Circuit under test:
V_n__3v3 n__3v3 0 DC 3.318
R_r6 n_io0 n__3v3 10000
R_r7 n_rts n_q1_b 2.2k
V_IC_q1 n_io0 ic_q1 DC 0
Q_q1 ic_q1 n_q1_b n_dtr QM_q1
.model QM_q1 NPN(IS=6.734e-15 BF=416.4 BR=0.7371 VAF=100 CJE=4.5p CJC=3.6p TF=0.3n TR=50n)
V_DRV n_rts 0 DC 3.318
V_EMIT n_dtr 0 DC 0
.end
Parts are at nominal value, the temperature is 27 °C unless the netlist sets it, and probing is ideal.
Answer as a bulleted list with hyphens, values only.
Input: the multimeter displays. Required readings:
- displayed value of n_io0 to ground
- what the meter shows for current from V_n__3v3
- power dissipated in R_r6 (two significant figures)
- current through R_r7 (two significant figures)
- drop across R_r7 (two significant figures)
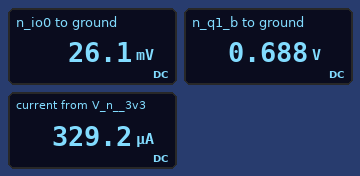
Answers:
- 26.1 mV
- 329.2 µA
- 1.1 mW
- 1.2 mA
- 2.6 V
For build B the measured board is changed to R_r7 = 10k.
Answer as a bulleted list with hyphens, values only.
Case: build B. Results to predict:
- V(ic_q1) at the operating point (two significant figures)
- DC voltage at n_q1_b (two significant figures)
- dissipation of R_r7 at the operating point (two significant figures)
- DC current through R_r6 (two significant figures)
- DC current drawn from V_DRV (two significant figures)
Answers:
- 36 mV
- 660 mV
- 710 µW
- 330 µA
- 270 µA
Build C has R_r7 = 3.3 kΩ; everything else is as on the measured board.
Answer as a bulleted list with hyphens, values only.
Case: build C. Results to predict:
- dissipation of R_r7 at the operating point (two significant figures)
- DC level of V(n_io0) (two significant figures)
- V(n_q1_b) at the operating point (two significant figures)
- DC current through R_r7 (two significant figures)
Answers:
- 2.1 mW
- 28 mV
- 680 mV
- 800 µA
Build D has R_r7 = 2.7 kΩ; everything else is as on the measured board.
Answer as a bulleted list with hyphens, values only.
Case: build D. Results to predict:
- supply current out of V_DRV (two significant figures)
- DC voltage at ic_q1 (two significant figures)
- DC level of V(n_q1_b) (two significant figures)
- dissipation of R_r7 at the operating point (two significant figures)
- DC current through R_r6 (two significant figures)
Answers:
- 980 µA
- 27 mV
- 680 mV
- 2.6 mW
- 330 µA
